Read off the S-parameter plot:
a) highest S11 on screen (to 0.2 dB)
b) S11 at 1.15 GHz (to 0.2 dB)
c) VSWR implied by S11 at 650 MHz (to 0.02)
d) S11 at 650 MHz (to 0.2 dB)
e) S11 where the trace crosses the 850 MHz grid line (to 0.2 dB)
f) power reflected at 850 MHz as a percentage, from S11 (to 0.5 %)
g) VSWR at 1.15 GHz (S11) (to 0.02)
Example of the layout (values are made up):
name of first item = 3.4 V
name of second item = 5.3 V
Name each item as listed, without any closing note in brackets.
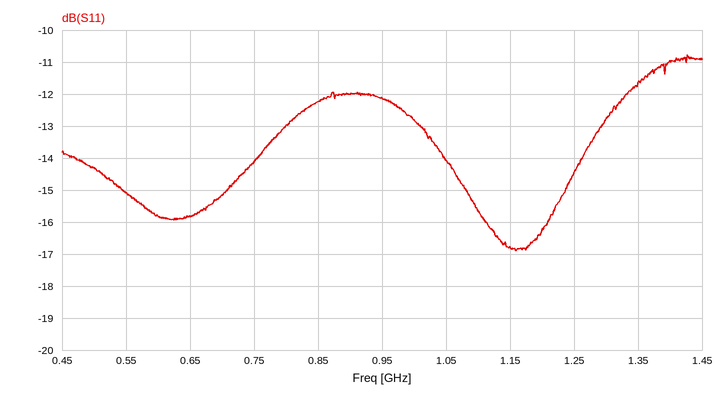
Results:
highest S11 on screen = -10.8 dB
S11 at 1.15 GHz = -16.8 dB
VSWR implied by S11 at 650 MHz = 1.38
S11 at 650 MHz = -15.8 dB
S11 where the trace crosses the 850 MHz grid line = -12.2 dB
power reflected at 850 MHz as a percentage, from S11 = 6.0 %
VSWR at 1.15 GHz (S11) = 1.34
